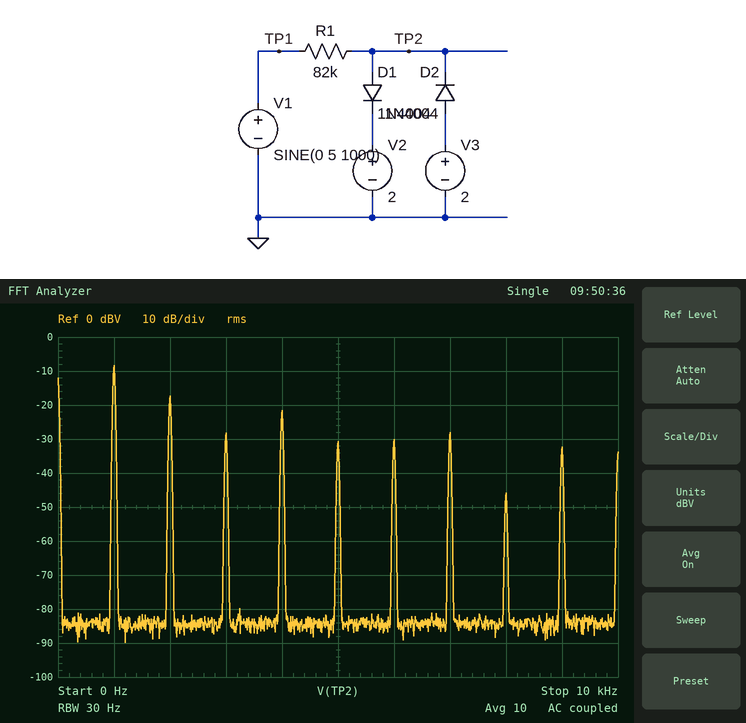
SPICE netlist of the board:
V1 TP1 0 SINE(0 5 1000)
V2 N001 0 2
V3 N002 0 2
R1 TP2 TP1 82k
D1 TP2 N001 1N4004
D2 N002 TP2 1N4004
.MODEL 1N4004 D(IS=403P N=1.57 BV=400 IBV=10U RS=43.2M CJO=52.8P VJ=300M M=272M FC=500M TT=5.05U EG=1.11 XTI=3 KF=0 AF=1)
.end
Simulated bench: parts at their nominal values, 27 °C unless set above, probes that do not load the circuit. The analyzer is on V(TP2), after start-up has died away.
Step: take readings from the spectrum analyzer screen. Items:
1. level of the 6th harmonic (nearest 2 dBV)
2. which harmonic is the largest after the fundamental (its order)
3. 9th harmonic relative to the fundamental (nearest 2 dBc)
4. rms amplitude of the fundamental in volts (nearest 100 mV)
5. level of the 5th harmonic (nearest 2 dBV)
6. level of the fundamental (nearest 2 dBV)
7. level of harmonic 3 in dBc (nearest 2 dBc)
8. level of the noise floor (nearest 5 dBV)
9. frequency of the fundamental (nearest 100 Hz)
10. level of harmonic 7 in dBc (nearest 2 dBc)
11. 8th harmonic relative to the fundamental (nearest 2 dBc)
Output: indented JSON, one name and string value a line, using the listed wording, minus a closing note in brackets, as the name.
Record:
{
  "level of the 6th harmonic": "-30 dBV",
  "which harmonic is the largest after the fundamental": "2",
  "9th harmonic relative to the fundamental": "-24 dBc",
  "rms amplitude of the fundamental in volts": "400 mV",
  "level of the 5th harmonic": "-30 dBV",
  "level of the fundamental": "-8 dBV",
  "level of harmonic 3 in dBc": "-20 dBc",
  "level of the noise floor": "-85 dBV",
  "frequency of the fundamental": "1.0 kHz",
  "level of harmonic 7 in dBc": "-20 dBc",
  "8th harmonic relative to the fundamental": "-38 dBc"
}
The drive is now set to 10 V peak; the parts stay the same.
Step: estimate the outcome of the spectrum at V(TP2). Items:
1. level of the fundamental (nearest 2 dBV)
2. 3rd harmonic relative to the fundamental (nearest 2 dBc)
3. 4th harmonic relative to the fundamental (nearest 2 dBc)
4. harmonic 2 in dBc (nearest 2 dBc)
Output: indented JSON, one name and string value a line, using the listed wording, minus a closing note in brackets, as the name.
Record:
{
  "level of the fundamental": "-8 dBV",
  "3rd harmonic relative to the fundamental": "-12 dBc",
  "4th harmonic relative to the fundamental": "-16 dBc",
  "harmonic 2 in dBc": "-14 dBc"
}
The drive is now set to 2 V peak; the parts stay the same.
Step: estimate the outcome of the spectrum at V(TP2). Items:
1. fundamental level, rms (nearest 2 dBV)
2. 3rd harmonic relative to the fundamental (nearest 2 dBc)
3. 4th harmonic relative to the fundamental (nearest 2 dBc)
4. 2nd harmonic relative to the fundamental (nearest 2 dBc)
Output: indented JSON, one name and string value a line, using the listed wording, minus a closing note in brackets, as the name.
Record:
{
  "fundamental level, rms": "-20 dBV",
  "3rd harmonic relative to the fundamental": "-8 dBc",
  "4th harmonic relative to the fundamental": "-12 dBc",
  "2nd harmonic relative to the fundamental": "-4 dBc"
}
